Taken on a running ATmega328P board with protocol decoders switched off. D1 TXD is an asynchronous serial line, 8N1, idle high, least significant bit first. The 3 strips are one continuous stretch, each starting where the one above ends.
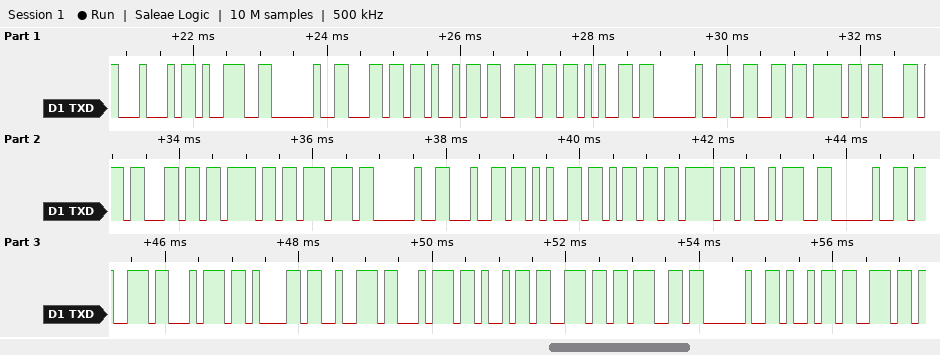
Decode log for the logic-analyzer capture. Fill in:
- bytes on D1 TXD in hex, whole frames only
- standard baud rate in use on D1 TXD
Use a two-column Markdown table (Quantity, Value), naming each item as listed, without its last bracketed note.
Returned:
| Quantity | Value |
|---|---|
| bytes on D1 TXD in hex, whole frames only | 0x44 0x39 0x20 0x6C 0x69 0x6E 0x65 0x20 0x66 0x6F 0x6C 0x6C 0x6F 0x77 0x20 0x64 0x65 0x6D 0x6F 0x3A 0x20 0x73 0x74 0x61 0x72 0x74 0x69 0x6E 0x67 0x20 0x69 0x6E |
| standard baud rate in use on D1 TXD | 9600 baud |
